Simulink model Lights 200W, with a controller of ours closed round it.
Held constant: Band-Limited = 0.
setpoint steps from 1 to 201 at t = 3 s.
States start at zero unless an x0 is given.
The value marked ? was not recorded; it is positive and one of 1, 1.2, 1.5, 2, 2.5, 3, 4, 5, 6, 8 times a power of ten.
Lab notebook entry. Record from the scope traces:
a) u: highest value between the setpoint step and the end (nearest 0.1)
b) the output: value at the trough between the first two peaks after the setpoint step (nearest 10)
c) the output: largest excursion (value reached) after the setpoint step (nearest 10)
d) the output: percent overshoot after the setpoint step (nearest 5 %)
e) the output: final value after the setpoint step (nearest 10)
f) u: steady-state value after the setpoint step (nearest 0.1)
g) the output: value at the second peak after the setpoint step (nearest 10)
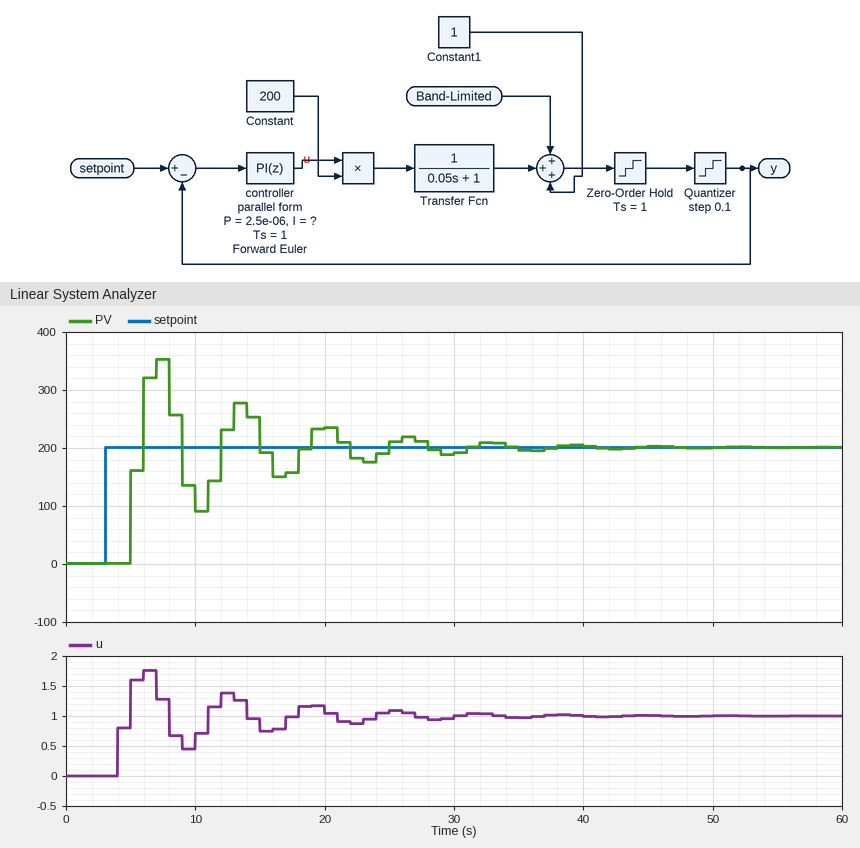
1.8
90
350
75 %
200
1.0
280
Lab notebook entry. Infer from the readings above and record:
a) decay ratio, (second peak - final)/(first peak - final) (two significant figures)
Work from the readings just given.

0.53
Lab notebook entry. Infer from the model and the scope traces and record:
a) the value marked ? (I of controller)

0.004
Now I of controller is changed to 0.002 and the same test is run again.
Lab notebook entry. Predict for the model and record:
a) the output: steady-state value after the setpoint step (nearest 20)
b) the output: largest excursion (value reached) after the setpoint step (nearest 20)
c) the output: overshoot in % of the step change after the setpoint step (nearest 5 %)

200
220
10 %
